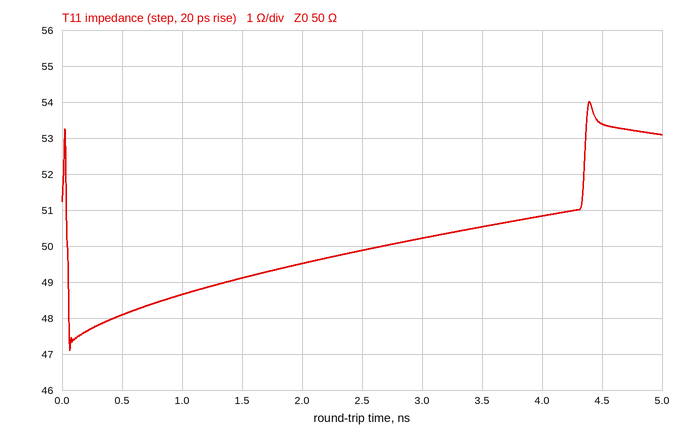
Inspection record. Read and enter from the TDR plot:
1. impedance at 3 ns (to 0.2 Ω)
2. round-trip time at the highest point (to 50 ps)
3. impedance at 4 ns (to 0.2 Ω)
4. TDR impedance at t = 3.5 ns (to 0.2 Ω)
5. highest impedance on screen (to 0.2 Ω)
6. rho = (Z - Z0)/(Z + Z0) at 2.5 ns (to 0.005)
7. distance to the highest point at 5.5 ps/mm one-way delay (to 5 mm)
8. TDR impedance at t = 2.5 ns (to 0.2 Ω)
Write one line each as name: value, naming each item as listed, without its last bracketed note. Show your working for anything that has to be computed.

impedance at 3 ns: 50.2 Ω
round-trip time at the highest point: 4.40 ns
impedance at 4 ns: 50.8 Ω
TDR impedance at t = 3.5 ns: 50.6 Ω
highest impedance on screen: 54.0 Ω
rho = (Z - Z0)/(Z + Z0) at 2.5 ns: (49.8 − 50)/(49.8 + 50) ≈ 0.000
distance to the highest point at 5.5 ps/mm one-way delay: 4.40 ns / 2 / 5.5 ps/mm ≈ 400 mm
TDR impedance at t = 2.5 ns: 49.8 Ω
